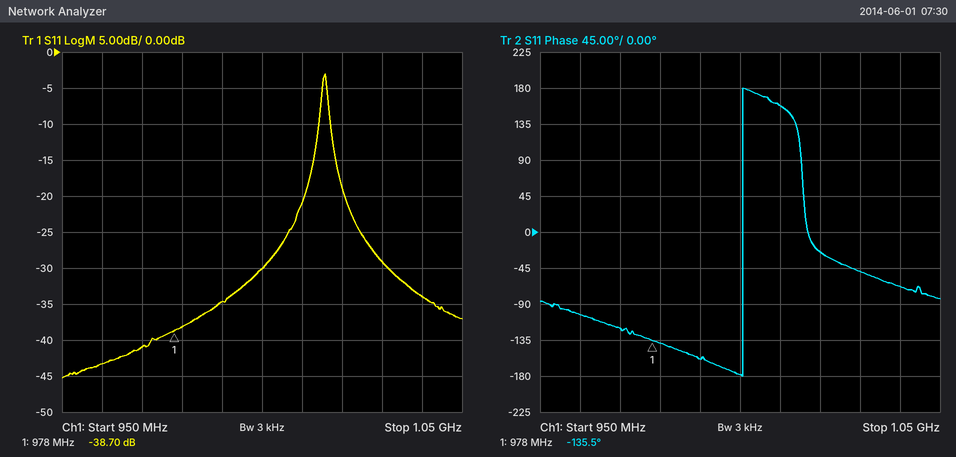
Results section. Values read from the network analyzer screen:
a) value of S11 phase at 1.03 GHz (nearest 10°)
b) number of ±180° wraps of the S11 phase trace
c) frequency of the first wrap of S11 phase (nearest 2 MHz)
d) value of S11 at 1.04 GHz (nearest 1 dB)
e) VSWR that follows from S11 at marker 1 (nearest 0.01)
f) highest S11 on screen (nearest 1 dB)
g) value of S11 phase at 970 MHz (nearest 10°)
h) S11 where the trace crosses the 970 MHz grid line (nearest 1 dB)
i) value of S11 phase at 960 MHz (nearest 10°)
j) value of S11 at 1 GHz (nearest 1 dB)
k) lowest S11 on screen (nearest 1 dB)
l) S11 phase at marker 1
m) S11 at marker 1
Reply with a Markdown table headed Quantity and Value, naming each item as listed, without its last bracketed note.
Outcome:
| Quantity | Value |
|---|---|
| value of S11 phase at 1.03 GHz | -50° |
| number of ±180° wraps of the S11 phase trace | 1 |
| frequency of the first wrap of S11 phase | 1.000 GHz |
| value of S11 at 1.04 GHz | -34 dB |
| VSWR that follows from S11 at marker 1 | 1.02 |
| highest S11 on screen | -3 dB |
| value of S11 phase at 970 MHz | -120° |
| S11 where the trace crosses the 970 MHz grid line | -41 dB |
| value of S11 phase at 960 MHz | -100° |
| value of S11 at 1 GHz | -30 dB |
| lowest S11 on screen | -45 dB |
| S11 phase at marker 1 | -135.5° |
| S11 at marker 1 | -38.70 dB |
